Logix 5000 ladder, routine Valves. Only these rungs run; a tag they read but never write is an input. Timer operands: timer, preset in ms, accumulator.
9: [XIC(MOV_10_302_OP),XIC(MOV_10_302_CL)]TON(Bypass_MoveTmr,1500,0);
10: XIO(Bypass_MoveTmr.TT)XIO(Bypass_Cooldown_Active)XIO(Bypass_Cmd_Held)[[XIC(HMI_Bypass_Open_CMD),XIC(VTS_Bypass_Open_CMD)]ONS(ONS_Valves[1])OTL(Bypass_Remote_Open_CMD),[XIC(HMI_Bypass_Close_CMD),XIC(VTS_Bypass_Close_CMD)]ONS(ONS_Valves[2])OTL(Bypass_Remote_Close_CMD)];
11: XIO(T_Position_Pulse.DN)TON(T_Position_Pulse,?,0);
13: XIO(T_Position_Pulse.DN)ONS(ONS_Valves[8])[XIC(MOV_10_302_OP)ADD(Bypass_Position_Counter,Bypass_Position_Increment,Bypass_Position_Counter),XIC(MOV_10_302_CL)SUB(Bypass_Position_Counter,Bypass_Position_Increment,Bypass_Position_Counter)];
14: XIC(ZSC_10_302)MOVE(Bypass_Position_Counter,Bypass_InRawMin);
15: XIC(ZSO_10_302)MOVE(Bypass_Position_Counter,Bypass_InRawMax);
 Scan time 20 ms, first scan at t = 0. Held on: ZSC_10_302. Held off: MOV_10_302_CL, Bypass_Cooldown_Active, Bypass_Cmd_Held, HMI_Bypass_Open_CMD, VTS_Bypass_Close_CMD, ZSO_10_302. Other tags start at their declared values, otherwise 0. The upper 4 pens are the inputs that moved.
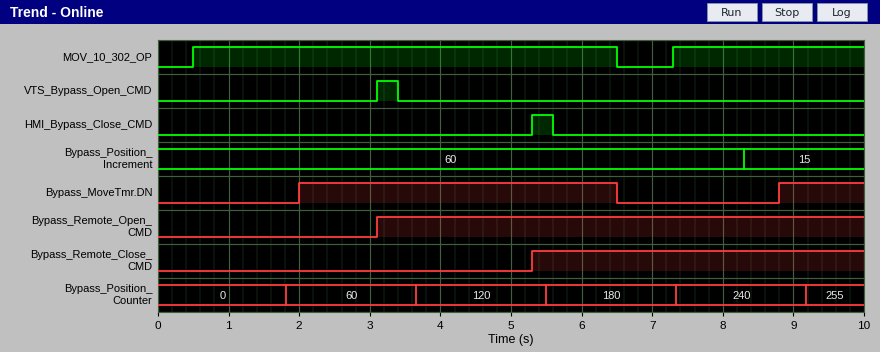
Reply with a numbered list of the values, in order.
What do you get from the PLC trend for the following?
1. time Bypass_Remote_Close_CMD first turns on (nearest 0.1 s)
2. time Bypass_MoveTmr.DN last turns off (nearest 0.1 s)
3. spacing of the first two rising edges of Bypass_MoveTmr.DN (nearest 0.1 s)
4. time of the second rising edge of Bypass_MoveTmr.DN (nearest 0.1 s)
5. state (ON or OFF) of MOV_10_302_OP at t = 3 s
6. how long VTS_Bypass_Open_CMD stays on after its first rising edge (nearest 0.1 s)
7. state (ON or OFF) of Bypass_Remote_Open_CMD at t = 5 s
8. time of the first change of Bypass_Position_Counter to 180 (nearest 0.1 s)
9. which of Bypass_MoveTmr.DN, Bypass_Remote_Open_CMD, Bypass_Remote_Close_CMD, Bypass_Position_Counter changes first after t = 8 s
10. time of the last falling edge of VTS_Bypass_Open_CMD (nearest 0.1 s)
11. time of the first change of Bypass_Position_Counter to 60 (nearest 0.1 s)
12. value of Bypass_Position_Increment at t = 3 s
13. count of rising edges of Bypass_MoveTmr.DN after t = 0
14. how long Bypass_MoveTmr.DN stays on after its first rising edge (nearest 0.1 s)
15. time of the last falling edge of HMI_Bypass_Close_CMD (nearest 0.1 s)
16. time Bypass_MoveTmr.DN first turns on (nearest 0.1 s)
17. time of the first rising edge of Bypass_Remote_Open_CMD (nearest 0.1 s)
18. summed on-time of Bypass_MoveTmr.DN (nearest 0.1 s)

1. 5.3 s
2. 6.5 s
3. 6.8 s
4. 8.8 s
5. ON
6. 0.3 s
7. ON
8. 5.5 s
9. Bypass_MoveTmr.DN
10. 3.4 s
11. 1.8 s
12. 60
13. 2
14. 4.5 s
15. 5.6 s
16. 2.0 s
17. 3.1 s
18. 5.7 s
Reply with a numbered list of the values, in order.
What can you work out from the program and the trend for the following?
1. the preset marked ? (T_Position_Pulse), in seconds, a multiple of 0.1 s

1. 1.8 s
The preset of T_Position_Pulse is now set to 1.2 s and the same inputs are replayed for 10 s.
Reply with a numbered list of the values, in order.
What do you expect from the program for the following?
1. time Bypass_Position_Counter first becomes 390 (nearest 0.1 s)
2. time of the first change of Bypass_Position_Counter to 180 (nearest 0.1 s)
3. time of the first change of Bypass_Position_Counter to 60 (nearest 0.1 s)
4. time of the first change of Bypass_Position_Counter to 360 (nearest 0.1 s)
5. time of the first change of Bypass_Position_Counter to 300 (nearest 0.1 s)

1. 9.9 s
2. 3.7 s
3. 1.2 s
4. 7.4 s
5. 6.2 s
